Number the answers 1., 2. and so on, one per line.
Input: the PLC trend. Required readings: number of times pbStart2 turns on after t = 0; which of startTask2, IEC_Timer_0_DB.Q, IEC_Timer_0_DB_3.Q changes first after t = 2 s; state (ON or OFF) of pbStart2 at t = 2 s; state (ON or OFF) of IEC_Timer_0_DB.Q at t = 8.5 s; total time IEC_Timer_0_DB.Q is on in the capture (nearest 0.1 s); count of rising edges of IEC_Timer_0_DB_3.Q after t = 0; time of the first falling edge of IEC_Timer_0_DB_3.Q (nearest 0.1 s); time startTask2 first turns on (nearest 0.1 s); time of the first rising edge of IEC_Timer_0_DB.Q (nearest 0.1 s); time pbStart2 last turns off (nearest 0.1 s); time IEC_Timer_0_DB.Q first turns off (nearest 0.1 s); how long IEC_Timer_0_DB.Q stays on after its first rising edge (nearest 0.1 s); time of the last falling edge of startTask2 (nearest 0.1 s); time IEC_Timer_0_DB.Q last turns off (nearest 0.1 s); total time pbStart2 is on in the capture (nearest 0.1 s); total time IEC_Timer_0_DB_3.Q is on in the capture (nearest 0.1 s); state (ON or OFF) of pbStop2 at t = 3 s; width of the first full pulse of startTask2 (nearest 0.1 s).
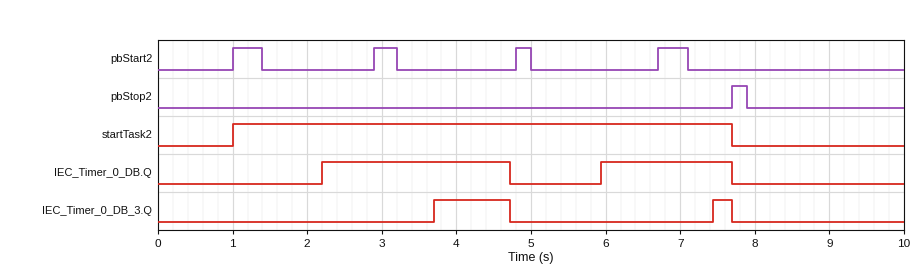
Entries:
1. 4
2. IEC_Timer_0_DB.Q
3. OFF
4. OFF
5. 4.3 s
6. 2
7. 4.7 s
8. 1.0 s
9. 2.2 s
10. 7.1 s
11. 4.7 s
12. 2.5 s
13. 7.7 s
14. 7.7 s
15. 1.3 s
16. 1.3 s
17. OFF
18. 6.7 s
